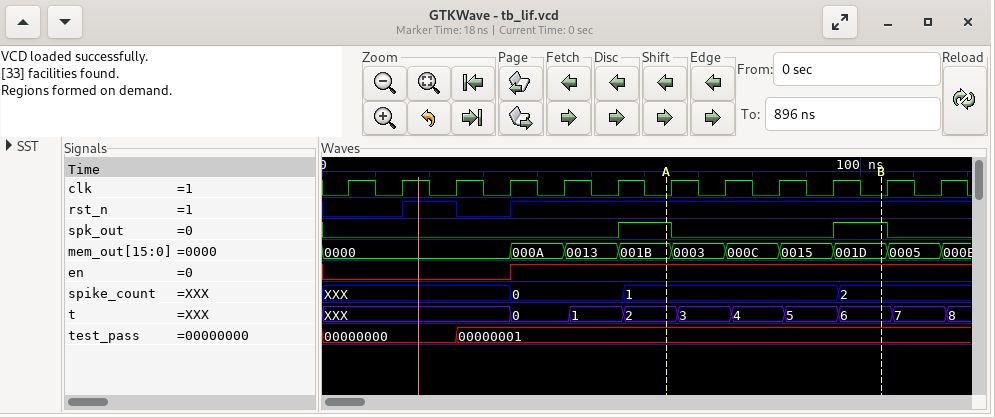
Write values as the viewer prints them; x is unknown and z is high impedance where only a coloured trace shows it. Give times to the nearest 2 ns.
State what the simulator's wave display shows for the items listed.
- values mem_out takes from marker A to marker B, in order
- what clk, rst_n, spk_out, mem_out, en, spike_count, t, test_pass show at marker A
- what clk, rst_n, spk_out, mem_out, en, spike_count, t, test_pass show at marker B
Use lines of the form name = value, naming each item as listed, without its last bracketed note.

values mem_out takes from marker A to marker B, in order = 001B, 0003, 000C, 0015, 001D
what clk, rst_n, spk_out, mem_out, en, spike_count, t, test_pass show at marker A = clk=0, rst_n=1, spk_out=1, mem_out=001B, en=1, spike_count=1, t=2, test_pass=00000001
what clk, rst_n, spk_out, mem_out, en, spike_count, t, test_pass show at marker B = clk=0, rst_n=1, spk_out=1, mem_out=001D, en=1, spike_count=2, t=6, test_pass=00000001
